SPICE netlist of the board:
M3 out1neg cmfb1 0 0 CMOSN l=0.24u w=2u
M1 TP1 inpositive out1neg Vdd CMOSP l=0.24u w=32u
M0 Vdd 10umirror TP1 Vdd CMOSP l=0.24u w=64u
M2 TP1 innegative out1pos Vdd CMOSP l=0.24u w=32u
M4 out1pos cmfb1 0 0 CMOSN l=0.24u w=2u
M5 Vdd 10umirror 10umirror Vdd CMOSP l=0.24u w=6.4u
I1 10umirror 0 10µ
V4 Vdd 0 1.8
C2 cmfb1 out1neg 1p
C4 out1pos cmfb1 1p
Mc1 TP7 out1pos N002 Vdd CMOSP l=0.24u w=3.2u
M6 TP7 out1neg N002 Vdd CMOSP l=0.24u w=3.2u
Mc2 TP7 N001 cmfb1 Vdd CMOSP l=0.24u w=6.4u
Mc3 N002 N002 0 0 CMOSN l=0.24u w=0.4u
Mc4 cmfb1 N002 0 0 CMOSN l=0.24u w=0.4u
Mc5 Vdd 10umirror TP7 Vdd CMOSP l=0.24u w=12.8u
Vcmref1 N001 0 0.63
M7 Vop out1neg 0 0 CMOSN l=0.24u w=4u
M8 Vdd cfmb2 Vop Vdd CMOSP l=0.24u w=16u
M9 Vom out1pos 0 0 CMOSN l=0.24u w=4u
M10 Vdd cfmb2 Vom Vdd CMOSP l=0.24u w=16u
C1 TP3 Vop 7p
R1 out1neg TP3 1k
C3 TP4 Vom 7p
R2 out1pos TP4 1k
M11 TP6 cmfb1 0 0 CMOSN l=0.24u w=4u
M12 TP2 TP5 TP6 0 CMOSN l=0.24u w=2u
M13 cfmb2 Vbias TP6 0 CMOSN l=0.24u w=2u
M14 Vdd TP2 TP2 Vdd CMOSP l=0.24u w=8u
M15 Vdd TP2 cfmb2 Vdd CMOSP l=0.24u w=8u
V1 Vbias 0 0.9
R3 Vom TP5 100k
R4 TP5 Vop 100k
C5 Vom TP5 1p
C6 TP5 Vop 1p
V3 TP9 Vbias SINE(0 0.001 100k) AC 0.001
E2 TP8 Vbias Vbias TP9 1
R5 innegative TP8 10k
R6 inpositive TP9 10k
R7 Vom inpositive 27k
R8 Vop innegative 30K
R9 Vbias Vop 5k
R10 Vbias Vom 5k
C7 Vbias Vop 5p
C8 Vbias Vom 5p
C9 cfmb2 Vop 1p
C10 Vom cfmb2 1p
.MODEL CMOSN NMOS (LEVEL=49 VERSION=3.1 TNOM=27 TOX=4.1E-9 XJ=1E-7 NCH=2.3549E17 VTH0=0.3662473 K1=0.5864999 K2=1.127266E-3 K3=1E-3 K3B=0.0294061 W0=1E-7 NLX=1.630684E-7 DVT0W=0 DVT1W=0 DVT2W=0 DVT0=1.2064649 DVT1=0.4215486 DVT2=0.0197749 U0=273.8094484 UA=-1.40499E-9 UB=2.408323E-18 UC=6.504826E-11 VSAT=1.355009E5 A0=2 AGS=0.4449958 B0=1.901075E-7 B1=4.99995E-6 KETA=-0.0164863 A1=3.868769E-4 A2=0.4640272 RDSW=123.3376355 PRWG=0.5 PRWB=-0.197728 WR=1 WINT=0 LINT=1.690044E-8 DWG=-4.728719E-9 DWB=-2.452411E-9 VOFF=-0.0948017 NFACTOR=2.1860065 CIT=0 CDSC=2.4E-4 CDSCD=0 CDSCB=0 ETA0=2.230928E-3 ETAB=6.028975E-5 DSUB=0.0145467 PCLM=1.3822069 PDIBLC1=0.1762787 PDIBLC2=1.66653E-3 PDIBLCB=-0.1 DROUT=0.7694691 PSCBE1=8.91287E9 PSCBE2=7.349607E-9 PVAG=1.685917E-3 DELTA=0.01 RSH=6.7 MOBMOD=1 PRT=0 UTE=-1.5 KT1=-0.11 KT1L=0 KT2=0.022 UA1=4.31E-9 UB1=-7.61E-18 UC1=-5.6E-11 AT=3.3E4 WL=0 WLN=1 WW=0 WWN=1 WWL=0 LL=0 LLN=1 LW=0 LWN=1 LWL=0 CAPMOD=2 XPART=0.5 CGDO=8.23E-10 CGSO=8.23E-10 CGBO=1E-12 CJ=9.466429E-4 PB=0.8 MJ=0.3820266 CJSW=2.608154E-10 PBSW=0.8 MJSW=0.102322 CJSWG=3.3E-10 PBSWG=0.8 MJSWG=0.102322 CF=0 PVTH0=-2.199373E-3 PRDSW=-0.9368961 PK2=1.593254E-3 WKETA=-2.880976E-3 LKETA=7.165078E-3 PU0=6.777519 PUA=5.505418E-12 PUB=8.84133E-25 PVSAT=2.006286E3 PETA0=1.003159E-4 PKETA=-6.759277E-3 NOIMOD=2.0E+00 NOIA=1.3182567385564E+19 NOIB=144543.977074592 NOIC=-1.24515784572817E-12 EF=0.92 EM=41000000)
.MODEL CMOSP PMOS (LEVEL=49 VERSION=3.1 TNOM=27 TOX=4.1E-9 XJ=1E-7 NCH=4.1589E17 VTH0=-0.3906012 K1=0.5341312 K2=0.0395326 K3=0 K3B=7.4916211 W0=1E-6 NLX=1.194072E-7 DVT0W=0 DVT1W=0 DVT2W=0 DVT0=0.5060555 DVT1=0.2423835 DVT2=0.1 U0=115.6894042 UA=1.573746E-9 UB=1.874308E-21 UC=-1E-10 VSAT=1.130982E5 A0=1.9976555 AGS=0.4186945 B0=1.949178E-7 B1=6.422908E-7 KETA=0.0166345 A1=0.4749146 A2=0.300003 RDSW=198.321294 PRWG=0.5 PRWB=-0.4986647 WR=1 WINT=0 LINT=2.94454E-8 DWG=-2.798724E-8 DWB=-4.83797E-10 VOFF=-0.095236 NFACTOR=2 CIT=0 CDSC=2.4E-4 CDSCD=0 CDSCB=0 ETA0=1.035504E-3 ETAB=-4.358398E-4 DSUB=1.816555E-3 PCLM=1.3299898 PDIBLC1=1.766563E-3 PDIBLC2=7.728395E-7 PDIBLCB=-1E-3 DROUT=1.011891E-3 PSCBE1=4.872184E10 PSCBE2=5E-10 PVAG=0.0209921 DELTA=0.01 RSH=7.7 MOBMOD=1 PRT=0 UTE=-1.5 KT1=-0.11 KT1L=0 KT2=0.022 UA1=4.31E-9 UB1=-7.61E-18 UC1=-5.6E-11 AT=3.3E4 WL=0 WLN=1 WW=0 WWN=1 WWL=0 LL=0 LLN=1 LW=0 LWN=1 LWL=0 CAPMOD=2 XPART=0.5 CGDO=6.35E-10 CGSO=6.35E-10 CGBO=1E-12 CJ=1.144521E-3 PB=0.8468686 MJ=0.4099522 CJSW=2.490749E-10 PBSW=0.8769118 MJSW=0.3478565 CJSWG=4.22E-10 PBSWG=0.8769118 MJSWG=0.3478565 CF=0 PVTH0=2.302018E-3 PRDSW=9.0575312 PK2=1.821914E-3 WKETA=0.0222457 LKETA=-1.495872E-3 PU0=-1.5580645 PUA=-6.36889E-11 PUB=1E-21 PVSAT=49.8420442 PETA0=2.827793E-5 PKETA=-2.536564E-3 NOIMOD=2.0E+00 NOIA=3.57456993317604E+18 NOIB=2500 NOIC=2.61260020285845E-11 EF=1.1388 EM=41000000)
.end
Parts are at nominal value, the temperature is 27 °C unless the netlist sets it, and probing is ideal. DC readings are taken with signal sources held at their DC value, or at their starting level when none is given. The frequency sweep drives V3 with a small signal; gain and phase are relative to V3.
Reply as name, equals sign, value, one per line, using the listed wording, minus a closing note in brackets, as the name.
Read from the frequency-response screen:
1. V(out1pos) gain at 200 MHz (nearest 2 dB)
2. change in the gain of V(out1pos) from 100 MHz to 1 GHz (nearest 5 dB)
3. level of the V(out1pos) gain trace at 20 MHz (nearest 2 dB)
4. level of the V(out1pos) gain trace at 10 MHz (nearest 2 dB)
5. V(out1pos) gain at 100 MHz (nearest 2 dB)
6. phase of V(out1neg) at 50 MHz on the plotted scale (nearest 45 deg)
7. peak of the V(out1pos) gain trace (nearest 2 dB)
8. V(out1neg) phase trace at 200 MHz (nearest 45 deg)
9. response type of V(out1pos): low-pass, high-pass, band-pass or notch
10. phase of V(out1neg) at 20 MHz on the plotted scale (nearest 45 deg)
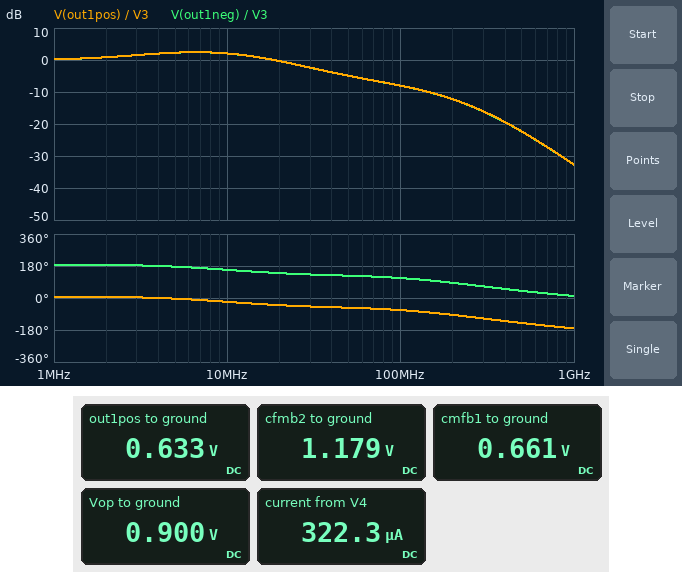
V(out1pos) gain at 200 MHz = -12 dB
change in the gain of V(out1pos) from 100 MHz to 1 GHz = -25 dB
level of the V(out1pos) gain trace at 20 MHz = 0 dB
level of the V(out1pos) gain trace at 10 MHz = 2 dB
V(out1pos) gain at 100 MHz = -8 dB
phase of V(out1neg) at 50 MHz on the plotted scale = 135 deg
peak of the V(out1pos) gain trace = 2 dB
V(out1neg) phase trace at 200 MHz = 90 deg
response type of V(out1pos): low-pass, high-pass, band-pass or notch = low-pass
phase of V(out1neg) at 20 MHz on the plotted scale = 135 deg
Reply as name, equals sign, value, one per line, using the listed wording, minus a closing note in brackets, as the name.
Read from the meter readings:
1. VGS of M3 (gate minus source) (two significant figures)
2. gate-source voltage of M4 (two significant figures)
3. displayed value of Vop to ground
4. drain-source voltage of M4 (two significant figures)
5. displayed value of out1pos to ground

VGS of M3 (gate minus source) = 660 mV
gate-source voltage of M4 = 660 mV
displayed value of Vop to ground = 0.900 V
drain-source voltage of M4 = 630 mV
displayed value of out1pos to ground = 0.633 V
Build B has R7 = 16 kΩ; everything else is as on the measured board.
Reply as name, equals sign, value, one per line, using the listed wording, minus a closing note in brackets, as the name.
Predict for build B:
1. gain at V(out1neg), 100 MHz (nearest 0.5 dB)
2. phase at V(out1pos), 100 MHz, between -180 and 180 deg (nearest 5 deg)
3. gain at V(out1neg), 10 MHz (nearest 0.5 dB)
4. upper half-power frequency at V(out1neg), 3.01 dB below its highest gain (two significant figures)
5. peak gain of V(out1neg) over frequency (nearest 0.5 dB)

gain at V(out1neg), 100 MHz = -8.5 dB
phase at V(out1pos), 100 MHz, between -180 and 180 deg = -65 deg
gain at V(out1neg), 10 MHz = 1.5 dB
upper half-power frequency at V(out1neg), 3.01 dB below its highest gain = 22 MHz
peak gain of V(out1neg) over frequency = 2.0 dB
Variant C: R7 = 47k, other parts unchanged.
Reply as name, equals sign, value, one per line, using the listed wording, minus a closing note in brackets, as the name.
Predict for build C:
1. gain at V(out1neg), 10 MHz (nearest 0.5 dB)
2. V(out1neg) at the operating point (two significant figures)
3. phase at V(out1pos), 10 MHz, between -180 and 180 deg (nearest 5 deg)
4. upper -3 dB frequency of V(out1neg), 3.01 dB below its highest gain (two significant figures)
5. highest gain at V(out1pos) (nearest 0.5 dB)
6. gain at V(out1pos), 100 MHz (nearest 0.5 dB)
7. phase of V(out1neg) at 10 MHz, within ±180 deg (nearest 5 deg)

gain at V(out1neg), 10 MHz = 2.5 dB
V(out1neg) at the operating point = 630 mV
phase at V(out1pos), 10 MHz, between -180 and 180 deg = -25 deg
upper -3 dB frequency of V(out1neg), 3.01 dB below its highest gain = 20 MHz
highest gain at V(out1pos) = 3.0 dB
gain at V(out1pos), 100 MHz = -7.5 dB
phase of V(out1neg) at 10 MHz, within ±180 deg = 155 deg
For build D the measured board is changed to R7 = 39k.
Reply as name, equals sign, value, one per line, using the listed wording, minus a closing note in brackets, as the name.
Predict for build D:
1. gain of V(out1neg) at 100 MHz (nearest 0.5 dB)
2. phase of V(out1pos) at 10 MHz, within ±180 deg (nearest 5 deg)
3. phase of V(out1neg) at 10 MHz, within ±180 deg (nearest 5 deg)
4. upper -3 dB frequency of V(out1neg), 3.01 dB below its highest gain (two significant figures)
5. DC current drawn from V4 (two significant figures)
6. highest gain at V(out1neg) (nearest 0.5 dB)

gain of V(out1neg) at 100 MHz = -7.5 dB
phase of V(out1pos) at 10 MHz, within ±180 deg = -25 deg
phase of V(out1neg) at 10 MHz, within ±180 deg = 155 deg
upper -3 dB frequency of V(out1neg), 3.01 dB below its highest gain = 20 MHz
DC current drawn from V4 = 320 µA
highest gain at V(out1neg) = 3.0 dB
